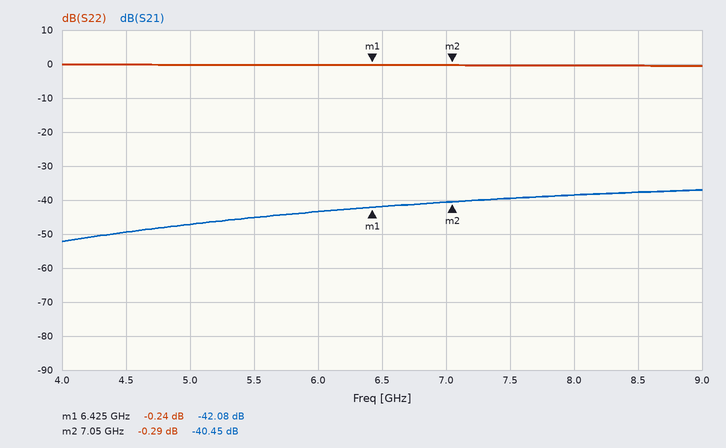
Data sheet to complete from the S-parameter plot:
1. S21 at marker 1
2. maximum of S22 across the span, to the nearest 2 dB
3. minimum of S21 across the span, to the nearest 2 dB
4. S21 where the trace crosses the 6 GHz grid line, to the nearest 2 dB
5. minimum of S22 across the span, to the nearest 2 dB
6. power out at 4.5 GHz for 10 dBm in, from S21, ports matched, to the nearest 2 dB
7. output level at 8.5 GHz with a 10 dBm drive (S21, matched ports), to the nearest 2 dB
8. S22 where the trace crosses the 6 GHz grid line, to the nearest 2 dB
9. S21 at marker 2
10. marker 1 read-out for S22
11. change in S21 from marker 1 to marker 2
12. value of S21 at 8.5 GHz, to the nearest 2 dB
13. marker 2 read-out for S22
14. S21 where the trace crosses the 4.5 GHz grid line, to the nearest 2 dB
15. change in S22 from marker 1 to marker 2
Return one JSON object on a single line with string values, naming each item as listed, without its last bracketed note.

{"S21 at marker 1": "-42.08 dB", "maximum of S22 across the span, to the nearest 2 dB": "0 dB", "minimum of S21 across the span, to the nearest 2 dB": "-52 dB", "S21 where the trace crosses the 6 GHz grid line, to the nearest 2 dB": "-44 dB", "minimum of S22 across the span, to the nearest 2 dB": "0 dB", "power out at 4.5 GHz for 10 dBm in, from S21, ports matched, to the nearest 2 dB": "-40 dBm", "output level at 8.5 GHz with a 10 dBm drive (S21, matched ports), to the nearest 2 dB": "-28 dBm", "S22 where the trace crosses the 6 GHz grid line, to the nearest 2 dB": "0 dB", "S21 at marker 2": "-40.45 dB", "marker 1 read-out for S22": "-0.24 dB", "change in S21 from marker 1 to marker 2": "1.63 dB", "value of S21 at 8.5 GHz, to the nearest 2 dB": "-38 dB", "marker 2 read-out for S22": "-0.29 dB", "S21 where the trace crosses the 4.5 GHz grid line, to the nearest 2 dB": "-50 dB", "change in S22 from marker 1 to marker 2": "-0.05 dB"}
